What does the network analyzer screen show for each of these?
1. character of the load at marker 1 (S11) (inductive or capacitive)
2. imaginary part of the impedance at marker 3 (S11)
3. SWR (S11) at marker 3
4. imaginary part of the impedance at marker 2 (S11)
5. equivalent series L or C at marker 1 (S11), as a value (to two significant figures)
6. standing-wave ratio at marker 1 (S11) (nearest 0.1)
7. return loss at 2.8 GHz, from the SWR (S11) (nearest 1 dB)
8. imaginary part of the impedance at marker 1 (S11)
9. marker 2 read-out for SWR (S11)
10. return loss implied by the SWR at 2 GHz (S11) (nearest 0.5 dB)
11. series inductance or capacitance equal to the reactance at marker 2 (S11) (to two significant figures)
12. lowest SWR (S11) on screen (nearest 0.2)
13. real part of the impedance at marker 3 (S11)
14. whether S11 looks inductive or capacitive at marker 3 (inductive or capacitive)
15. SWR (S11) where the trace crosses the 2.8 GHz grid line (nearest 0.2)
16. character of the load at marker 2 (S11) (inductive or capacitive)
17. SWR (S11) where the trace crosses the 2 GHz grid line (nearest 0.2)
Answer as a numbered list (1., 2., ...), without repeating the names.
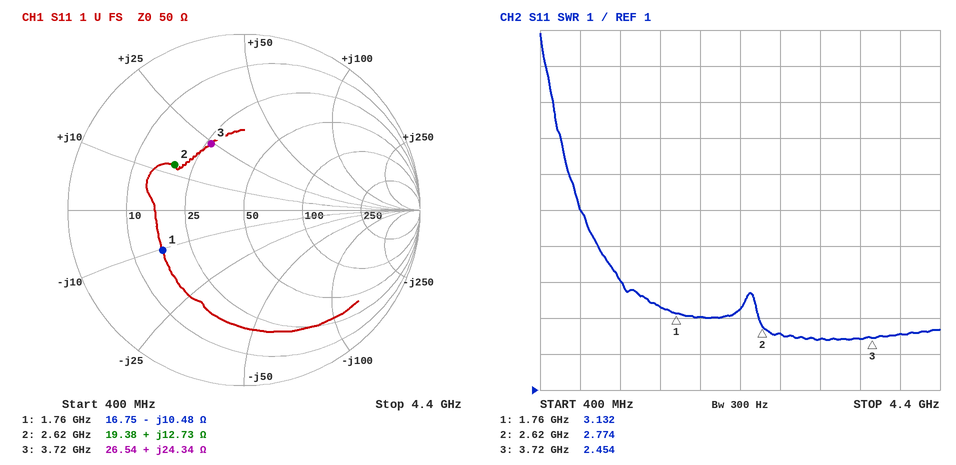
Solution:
1. capacitive
2. +24.34 Ω
3. 2.454
4. +12.73 Ω
5. 8.6 pF
6. 3.1
7. 7 dB
8. -10.48 Ω
9. 2.774
10. 6.0 dB
11. 770 pH
12. 2.4
13. 26.54 Ω
14. inductive
15. 2.6
16. inductive
17. 3.0
